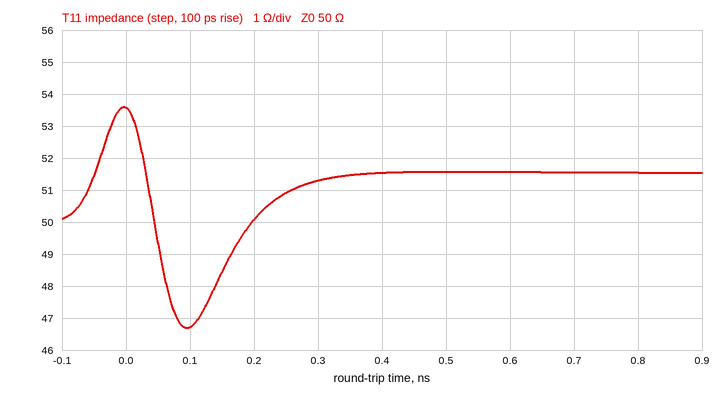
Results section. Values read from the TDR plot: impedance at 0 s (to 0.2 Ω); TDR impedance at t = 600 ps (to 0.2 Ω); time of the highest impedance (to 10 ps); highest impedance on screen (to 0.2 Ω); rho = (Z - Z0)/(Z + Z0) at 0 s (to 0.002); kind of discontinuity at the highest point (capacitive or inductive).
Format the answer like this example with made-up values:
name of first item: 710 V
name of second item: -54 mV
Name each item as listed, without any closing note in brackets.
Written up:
impedance at 0 s: 53.6 Ω
TDR impedance at t = 600 ps: 51.6 Ω
time of the highest impedance: 0 ps
highest impedance on screen: 53.6 Ω
rho = (Z - Z0)/(Z + Z0) at 0 s: +0.034
kind of discontinuity at the highest point: inductive
